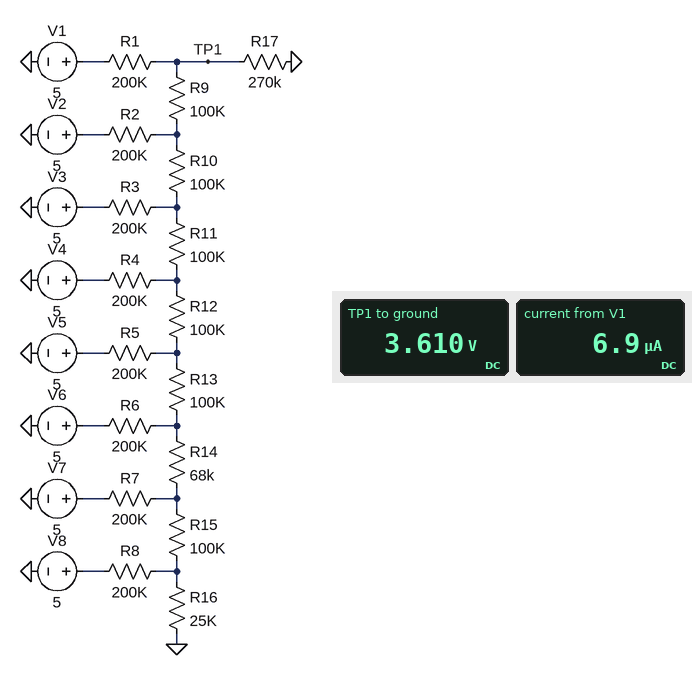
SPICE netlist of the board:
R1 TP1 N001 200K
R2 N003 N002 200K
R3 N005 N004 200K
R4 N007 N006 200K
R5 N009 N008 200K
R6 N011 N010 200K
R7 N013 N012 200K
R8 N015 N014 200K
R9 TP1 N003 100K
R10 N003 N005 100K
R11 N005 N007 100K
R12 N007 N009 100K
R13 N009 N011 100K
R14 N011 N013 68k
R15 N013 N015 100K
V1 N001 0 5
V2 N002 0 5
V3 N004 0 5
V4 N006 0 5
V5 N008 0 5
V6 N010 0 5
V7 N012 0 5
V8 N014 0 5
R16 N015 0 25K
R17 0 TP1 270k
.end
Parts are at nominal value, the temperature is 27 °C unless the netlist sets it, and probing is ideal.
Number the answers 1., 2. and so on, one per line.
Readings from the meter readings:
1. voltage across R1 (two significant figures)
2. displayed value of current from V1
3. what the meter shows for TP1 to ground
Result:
1. 1.4 V
2. 6.9 µA
3. 3.610 V
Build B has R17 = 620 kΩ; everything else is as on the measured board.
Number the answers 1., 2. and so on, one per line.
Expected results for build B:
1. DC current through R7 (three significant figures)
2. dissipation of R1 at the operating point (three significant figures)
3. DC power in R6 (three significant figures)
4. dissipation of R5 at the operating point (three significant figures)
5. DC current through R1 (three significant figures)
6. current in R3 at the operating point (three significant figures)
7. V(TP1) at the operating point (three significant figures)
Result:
1. 9.55 µA
2. 2.74 µW
3. 6.62 µW
4. 1.85 µW
5. 3.70 µA
6. 1.59 µA
7. 4.26 V
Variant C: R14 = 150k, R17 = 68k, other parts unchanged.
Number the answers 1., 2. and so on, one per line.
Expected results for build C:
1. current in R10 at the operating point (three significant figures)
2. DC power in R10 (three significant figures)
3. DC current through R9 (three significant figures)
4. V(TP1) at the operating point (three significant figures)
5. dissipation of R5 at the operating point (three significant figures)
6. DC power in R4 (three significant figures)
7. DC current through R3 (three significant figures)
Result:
1. 6.88 µA
2. 4.74 µW
3. 14.6 µA
4. 2.01 V
5. 1.86 µW
6. 1.70 µW
7. 4.24 µA
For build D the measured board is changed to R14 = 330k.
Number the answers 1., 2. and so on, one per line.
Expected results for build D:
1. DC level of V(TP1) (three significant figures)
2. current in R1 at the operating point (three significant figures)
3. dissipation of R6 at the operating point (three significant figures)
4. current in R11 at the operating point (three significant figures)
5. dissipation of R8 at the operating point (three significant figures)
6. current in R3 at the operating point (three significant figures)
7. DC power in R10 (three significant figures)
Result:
1. 3.63 V
2. 6.85 µA
3. 1.78 µW
4. 999 nA
5. 82.6 µW
6. 2.04 µA
7. 922 nW
